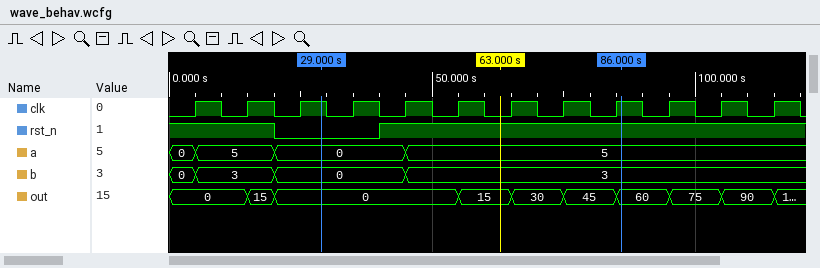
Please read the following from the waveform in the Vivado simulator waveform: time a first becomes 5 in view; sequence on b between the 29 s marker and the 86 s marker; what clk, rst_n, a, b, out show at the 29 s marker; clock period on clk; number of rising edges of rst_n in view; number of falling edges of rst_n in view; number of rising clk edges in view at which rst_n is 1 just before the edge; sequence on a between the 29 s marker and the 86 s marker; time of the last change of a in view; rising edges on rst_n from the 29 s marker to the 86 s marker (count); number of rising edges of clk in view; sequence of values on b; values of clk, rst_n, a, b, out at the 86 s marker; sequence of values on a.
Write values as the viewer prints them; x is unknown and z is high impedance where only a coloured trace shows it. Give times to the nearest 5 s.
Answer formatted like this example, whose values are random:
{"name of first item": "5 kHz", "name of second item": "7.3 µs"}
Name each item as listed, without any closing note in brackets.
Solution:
{"time a first becomes 5 in view": "5 s", "sequence on b between the 29 s marker and the 86 s marker": "0, 3", "what clk, rst_n, a, b, out show at the 29 s marker": "clk=1, rst_n=0, a=0, b=0, out=0", "clock period on clk": "10 s", "number of rising edges of rst_n in view": "1", "number of falling edges of rst_n in view": "1", "number of rising clk edges in view at which rst_n is 1 just before the edge": "10", "sequence on a between the 29 s marker and the 86 s marker": "0, 5", "time of the last change of a in view": "45 s", "rising edges on rst_n from the 29 s marker to the 86 s marker": "1", "number of rising edges of clk in view": "12", "sequence of values on b": "0, 3, 0, 3", "values of clk, rst_n, a, b, out at the 86 s marker": "clk=1, rst_n=1, a=5, b=3, out=60", "sequence of values on a": "0, 5, 0, 5"}
